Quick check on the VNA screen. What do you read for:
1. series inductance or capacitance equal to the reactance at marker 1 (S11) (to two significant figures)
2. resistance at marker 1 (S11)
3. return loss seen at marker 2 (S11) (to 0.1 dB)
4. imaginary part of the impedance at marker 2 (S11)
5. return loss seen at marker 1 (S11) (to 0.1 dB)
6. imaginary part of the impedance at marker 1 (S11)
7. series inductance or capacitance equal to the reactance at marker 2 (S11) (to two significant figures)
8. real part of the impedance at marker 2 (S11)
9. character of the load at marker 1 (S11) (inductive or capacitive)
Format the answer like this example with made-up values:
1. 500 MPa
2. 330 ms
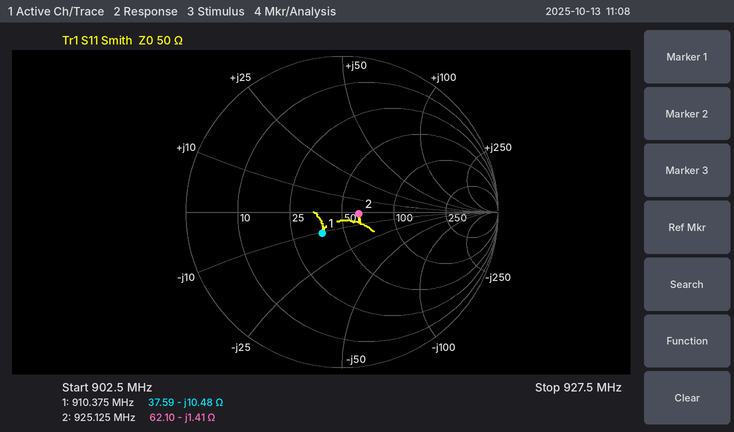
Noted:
1. 17 pF
2. 37.59 Ω
3. 19.3 dB
4. -1.41 Ω
5. 14.7 dB
6. -10.48 Ω
7. 120 pF
8. 62.10 Ω
9. capacitive
